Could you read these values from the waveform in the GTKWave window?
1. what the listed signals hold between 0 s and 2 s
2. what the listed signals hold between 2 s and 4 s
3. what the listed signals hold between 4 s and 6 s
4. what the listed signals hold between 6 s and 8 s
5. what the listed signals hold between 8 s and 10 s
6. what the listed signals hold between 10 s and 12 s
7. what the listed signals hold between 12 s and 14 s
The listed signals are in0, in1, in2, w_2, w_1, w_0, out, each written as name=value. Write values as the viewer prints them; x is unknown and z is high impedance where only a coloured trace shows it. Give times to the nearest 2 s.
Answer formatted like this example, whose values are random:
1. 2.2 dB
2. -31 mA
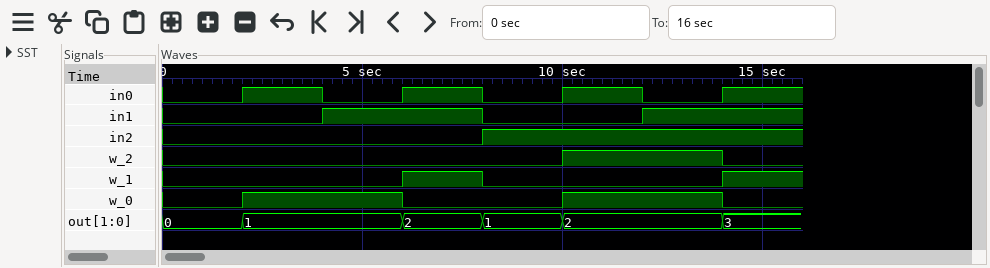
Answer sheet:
1. in0=0, in1=0, in2=0, w_2=0, w_1=0, w_0=0, out=0
2. in0=1, in1=0, in2=0, w_2=0, w_1=0, w_0=1, out=1
3. in0=0, in1=1, in2=0, w_2=0, w_1=0, w_0=1, out=1
4. in0=1, in1=1, in2=0, w_2=0, w_1=1, w_0=0, out=2
5. in0=0, in1=0, in2=1, w_2=0, w_1=0, w_0=0, out=1
6. in0=1, in1=0, in2=1, w_2=1, w_1=0, w_0=1, out=2
7. in0=0, in1=1, in2=1, w_2=1, w_1=0, w_0=1, out=2
